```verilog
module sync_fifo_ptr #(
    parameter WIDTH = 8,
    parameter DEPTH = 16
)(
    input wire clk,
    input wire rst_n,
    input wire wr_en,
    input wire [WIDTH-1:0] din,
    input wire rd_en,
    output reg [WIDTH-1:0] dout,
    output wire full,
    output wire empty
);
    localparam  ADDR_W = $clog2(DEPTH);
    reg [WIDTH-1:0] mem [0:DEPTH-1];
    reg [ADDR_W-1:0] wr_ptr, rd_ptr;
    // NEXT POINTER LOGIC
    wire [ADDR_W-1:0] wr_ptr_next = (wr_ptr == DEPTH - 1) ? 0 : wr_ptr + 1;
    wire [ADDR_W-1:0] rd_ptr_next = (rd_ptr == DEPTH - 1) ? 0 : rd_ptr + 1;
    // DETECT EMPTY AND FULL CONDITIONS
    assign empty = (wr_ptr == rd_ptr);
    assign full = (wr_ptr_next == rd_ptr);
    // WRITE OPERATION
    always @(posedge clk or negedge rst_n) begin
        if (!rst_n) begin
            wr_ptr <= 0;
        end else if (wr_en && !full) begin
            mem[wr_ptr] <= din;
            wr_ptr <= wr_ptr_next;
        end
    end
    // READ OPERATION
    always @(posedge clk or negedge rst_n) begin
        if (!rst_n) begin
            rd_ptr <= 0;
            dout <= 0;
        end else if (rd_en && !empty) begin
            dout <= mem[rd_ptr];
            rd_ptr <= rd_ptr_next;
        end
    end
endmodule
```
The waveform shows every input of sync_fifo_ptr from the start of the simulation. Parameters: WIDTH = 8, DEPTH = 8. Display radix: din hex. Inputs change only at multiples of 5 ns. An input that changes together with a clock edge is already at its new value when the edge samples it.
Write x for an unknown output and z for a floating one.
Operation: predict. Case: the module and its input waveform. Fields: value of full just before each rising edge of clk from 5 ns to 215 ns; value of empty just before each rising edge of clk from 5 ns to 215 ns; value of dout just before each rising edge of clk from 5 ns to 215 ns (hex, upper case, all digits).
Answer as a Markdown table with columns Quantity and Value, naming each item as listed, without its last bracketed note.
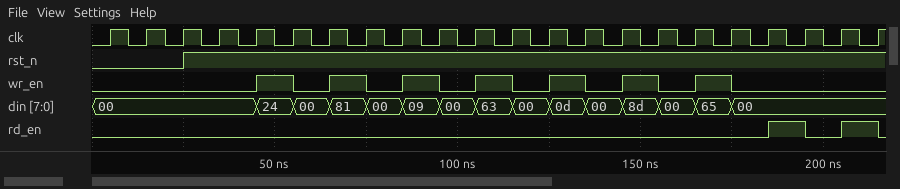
| Quantity | Value |
|---|---|
| value of full just before each rising edge of clk from 5 ns to 215 ns | 0 0 0 0 0 0 0 0 0 0 0 0 0 0 0 0 0 1 1 0 0 0 |
| value of empty just before each rising edge of clk from 5 ns to 215 ns | 1 1 1 1 1 0 0 0 0 0 0 0 0 0 0 0 0 0 0 0 0 0 |
| value of dout just before each rising edge of clk from 5 ns to 215 ns | 00, 00, 00, 00, 00, 00, 00, 00, 00, 00, 00, 00, 00, 00, 00, 00, 00, 00, 00, 24, 24, 81 |
